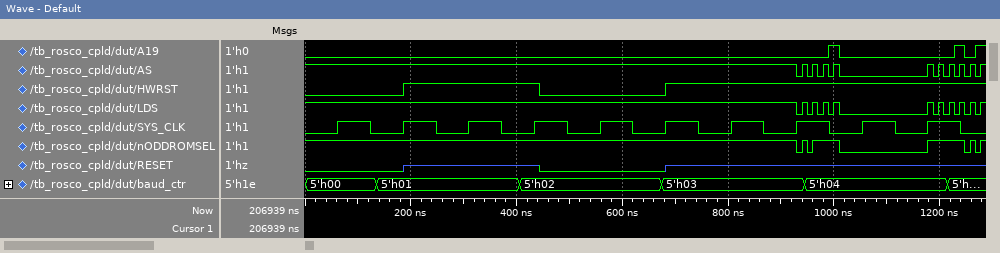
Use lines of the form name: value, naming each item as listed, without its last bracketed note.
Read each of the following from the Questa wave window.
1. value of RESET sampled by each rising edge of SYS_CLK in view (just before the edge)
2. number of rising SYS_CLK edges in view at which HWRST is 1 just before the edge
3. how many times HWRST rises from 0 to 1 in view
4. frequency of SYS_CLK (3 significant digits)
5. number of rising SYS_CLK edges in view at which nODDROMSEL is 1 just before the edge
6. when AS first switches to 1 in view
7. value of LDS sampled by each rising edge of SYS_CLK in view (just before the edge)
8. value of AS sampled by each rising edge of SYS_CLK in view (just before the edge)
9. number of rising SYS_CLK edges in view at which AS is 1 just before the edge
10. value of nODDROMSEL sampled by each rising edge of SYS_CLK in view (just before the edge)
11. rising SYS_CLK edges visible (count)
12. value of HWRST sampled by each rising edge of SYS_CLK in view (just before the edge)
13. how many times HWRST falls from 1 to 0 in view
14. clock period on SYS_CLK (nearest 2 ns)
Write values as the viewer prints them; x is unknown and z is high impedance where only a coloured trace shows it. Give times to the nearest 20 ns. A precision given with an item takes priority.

value of RESET sampled by each rising edge of SYS_CLK in view: 0 0 z z 0 0 z z z z
number of rising SYS_CLK edges in view at which HWRST is 1 just before the edge: 6
how many times HWRST rises from 0 to 1 in view: 2
frequency of SYS_CLK: 8.06 MHz
number of rising SYS_CLK edges in view at which nODDROMSEL is 1 just before the edge: 8
when AS first switches to 1 in view: 940 ns
value of LDS sampled by each rising edge of SYS_CLK in view: 1 1 1 1 1 1 1 1 0 0
value of AS sampled by each rising edge of SYS_CLK in view: 1 1 1 1 1 1 1 1 0 0
number of rising SYS_CLK edges in view at which AS is 1 just before the edge: 8
value of nODDROMSEL sampled by each rising edge of SYS_CLK in view: 1 1 1 1 1 1 1 1 0 0
rising SYS_CLK edges visible: 10
value of HWRST sampled by each rising edge of SYS_CLK in view: 0 0 1 1 0 0 1 1 1 1
how many times HWRST falls from 1 to 0 in view: 1
clock period on SYS_CLK: 124 ns
